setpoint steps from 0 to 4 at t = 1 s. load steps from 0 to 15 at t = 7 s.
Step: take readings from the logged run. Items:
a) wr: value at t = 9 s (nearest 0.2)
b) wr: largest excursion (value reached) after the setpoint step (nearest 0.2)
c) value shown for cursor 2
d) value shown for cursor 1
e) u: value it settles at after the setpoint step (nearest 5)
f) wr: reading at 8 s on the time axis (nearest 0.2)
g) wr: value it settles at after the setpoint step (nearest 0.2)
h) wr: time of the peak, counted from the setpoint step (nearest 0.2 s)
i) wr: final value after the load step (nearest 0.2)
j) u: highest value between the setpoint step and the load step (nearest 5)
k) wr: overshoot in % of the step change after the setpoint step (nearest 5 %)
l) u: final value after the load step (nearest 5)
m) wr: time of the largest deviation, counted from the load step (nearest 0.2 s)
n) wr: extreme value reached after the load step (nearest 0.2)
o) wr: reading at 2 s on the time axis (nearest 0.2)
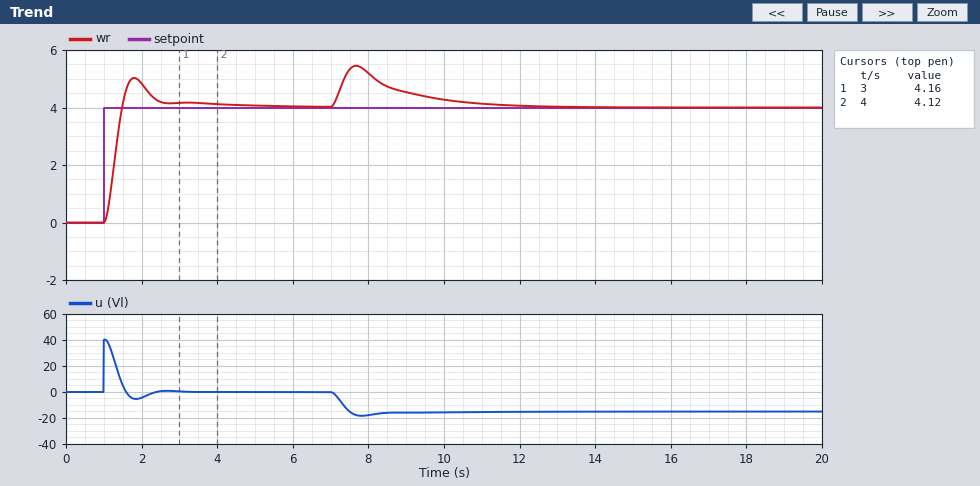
4.6
5.0
4.12
4.16
0
5.2
4.0
0.8 s
4.0
40
25 %
-15
0.6 s
5.4
4.8
